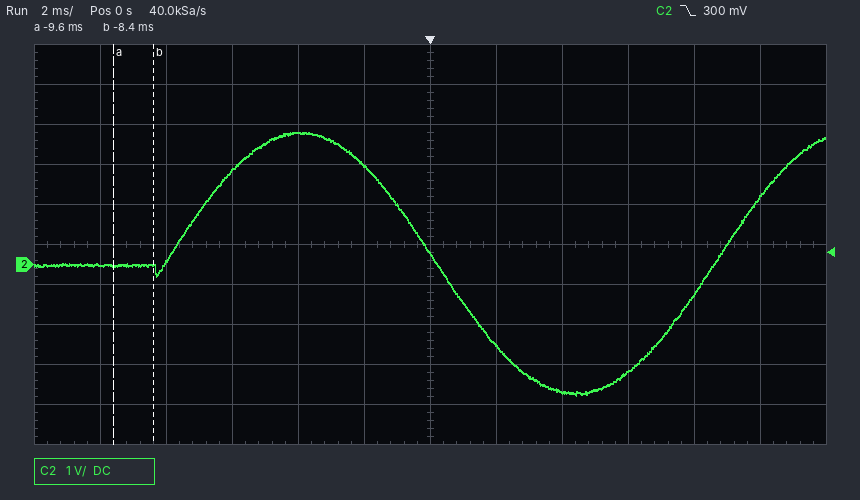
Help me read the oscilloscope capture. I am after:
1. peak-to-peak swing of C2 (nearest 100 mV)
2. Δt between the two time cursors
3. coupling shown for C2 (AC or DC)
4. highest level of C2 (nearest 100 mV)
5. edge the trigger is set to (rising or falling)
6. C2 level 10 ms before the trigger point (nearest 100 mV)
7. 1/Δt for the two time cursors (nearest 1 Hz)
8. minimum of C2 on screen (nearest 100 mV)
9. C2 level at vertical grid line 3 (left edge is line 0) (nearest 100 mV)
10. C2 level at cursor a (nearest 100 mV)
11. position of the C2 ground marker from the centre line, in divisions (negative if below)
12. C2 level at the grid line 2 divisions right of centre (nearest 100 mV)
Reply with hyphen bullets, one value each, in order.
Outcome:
- 6.6 V
- 1.2 ms
- DC
- 3.3 V
- falling
- 0.0 V
- 833 Hz
- -3.3 V
- 2.3 V
- 0.0 V
- -0.5 div
- -3.2 V
